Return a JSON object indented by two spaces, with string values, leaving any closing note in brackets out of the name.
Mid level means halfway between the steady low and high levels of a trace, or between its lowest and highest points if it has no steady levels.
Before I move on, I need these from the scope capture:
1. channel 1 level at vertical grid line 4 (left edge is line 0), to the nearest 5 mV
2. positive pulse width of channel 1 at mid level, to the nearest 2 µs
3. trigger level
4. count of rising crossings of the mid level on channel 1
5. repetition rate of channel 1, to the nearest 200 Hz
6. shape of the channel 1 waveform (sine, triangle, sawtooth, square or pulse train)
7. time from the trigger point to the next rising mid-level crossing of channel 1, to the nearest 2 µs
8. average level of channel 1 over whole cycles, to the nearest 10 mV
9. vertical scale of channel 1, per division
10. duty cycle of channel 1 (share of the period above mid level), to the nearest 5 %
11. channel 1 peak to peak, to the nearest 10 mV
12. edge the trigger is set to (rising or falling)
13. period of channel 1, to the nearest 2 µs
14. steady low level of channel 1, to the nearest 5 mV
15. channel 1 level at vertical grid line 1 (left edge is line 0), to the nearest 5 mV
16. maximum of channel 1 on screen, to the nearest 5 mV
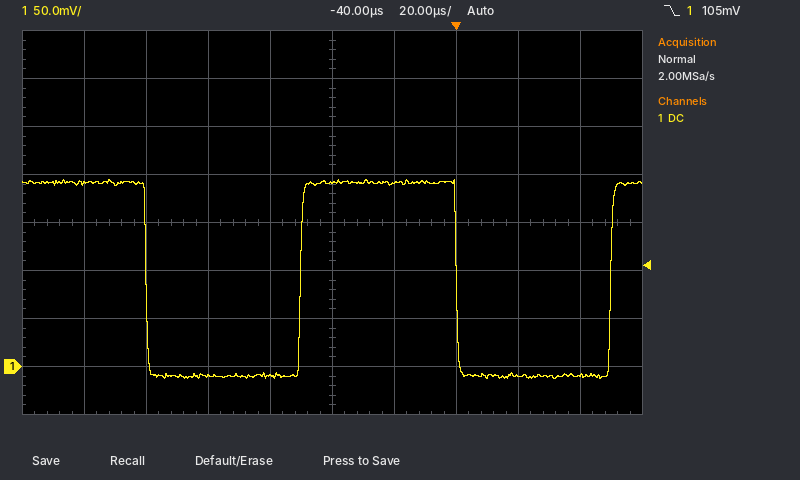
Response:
{
  "channel 1 level at vertical grid line 4 (left edge is line 0), to the nearest 5 mV": "-10 mV",
  "positive pulse width of channel 1 at mid level, to the nearest 2 µs": "50 µs",
  "trigger level": "105 mV",
  "count of rising crossings of the mid level on channel 1": "2",
  "repetition rate of channel 1, to the nearest 200 Hz": "10.0 kHz",
  "shape of the channel 1 waveform": "square",
  "time from the trigger point to the next rising mid-level crossing of channel 1, to the nearest 2 µs": "50 µs",
  "average level of channel 1 over whole cycles, to the nearest 10 mV": "90 mV",
  "vertical scale of channel 1, per division": "50 mV",
  "duty cycle of channel 1 (share of the period above mid level), to the nearest 5 %": "50 %",
  "channel 1 peak to peak, to the nearest 10 mV": "210 mV",
  "edge the trigger is set to": "falling",
  "period of channel 1, to the nearest 2 µs": "100 µs",
  "steady low level of channel 1, to the nearest 5 mV": "-10 mV",
  "channel 1 level at vertical grid line 1 (left edge is line 0), to the nearest 5 mV": "190 mV",
  "maximum of channel 1 on screen, to the nearest 5 mV": "195 mV"
}
